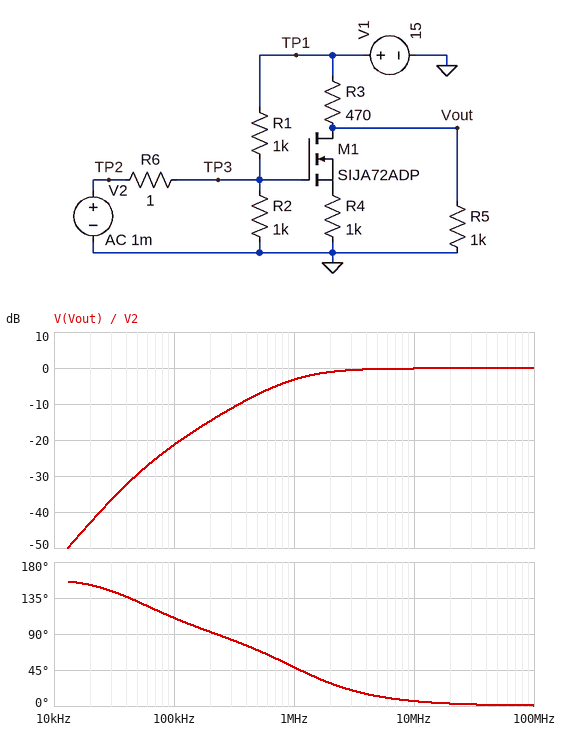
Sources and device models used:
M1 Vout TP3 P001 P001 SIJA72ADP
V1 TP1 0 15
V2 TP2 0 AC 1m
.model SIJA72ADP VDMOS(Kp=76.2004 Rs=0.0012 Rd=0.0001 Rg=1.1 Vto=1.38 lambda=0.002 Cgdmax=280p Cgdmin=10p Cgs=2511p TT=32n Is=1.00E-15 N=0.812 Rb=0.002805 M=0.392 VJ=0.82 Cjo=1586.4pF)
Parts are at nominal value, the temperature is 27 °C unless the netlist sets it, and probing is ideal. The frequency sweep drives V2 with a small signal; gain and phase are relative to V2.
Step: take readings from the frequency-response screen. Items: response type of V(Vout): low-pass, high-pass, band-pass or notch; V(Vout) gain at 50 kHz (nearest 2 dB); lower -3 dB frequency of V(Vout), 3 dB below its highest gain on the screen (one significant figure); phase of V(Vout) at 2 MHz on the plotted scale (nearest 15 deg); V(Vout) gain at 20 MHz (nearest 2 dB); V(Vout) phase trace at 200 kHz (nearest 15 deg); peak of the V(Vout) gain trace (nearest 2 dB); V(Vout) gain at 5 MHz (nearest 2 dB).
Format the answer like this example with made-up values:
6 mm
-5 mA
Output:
high-pass
-30 dB
1 MHz
30 deg
0 dB
90 deg
0 dB
0 dB
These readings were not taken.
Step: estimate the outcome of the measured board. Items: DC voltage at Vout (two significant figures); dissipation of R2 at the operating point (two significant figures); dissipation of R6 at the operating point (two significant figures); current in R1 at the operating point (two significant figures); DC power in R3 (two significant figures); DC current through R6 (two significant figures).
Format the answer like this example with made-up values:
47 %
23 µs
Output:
10 V
220 nW
220 µW
15 mA
49 mW
15 mA
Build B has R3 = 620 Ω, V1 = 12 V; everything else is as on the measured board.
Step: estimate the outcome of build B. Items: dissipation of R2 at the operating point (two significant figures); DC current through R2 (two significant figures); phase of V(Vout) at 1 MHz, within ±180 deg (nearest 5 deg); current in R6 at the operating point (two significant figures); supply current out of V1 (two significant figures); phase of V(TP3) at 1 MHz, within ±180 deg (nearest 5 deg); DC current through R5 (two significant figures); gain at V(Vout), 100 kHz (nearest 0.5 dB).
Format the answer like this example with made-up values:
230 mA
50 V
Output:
140 nW
12 µA
40 deg
12 mA
19 mA
0 deg
7.4 mA
-19.0 dB
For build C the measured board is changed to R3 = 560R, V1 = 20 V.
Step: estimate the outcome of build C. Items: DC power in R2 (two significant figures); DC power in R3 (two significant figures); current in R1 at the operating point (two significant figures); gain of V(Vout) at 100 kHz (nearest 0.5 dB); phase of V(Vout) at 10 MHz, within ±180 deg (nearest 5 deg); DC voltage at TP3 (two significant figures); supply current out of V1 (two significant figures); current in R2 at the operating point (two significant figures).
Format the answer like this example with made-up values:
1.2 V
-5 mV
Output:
400 nW
92 mW
20 mA
-21.0 dB
5 deg
20 mV
33 mA
20 µA
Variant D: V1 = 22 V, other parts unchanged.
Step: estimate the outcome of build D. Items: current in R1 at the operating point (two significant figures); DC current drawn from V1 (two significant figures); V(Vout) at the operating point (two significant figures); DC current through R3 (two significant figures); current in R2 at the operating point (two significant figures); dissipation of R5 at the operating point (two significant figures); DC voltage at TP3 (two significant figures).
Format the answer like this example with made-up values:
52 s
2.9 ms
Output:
22 mA
37 mA
15 V
15 mA
22 µA
220 mW
22 mV
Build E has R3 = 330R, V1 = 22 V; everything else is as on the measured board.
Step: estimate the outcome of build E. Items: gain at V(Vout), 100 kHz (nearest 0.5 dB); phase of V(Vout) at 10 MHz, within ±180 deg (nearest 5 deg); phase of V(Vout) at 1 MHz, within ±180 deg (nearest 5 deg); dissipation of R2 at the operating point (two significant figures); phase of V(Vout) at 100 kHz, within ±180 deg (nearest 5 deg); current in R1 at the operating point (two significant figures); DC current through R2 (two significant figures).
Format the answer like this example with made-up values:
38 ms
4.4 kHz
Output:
-25.0 dB
10 deg
60 deg
480 nW
115 deg
22 mA
22 µA
